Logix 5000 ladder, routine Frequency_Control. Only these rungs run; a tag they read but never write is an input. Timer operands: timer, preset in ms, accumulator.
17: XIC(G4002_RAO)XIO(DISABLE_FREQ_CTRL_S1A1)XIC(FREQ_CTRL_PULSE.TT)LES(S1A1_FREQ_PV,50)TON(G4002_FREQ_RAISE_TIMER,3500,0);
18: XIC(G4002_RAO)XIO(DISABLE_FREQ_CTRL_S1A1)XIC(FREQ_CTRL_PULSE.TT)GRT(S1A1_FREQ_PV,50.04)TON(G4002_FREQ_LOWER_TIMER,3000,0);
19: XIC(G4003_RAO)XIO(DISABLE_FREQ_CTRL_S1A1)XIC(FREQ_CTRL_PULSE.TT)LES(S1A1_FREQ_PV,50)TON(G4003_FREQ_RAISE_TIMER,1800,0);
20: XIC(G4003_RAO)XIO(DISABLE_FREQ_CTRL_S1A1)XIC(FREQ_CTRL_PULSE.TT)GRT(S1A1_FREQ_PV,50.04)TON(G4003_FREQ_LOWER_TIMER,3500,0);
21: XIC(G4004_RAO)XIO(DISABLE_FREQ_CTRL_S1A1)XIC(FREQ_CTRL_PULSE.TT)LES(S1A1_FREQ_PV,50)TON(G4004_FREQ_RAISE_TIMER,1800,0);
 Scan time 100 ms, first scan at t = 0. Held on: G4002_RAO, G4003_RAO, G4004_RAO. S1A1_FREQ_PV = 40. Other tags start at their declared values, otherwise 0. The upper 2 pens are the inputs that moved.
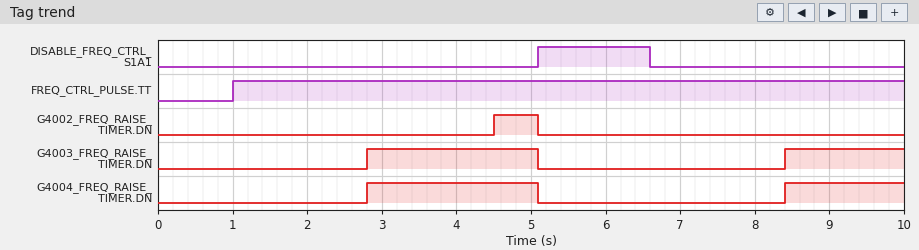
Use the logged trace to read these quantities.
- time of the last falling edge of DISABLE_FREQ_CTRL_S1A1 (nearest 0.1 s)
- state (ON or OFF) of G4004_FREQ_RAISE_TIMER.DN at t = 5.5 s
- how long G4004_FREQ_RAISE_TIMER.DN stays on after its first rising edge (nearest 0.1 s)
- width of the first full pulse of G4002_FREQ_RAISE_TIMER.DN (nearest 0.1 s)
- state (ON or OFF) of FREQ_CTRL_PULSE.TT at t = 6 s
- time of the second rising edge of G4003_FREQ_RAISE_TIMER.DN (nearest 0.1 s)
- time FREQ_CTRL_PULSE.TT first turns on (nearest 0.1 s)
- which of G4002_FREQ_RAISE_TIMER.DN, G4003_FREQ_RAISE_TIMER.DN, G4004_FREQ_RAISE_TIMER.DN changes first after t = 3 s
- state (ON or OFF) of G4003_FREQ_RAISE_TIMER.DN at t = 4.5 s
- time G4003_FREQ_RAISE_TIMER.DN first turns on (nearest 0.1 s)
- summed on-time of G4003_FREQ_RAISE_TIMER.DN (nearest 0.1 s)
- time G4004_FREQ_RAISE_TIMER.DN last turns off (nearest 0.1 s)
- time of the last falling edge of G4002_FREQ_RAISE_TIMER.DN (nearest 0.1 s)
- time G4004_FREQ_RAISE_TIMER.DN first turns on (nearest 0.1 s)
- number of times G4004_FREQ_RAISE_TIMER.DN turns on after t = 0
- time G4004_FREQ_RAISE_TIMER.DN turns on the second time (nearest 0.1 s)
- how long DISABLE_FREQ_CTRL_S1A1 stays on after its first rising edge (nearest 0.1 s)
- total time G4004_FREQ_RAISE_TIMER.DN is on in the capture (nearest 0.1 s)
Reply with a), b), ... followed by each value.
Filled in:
a) 6.6 s
b) OFF
c) 2.3 s
d) 0.6 s
e) ON
f) 8.4 s
g) 1.0 s
h) G4002_FREQ_RAISE_TIMER.DN
i) ON
j) 2.8 s
k) 3.9 s
l) 5.1 s
m) 5.1 s
n) 2.8 s
o) 2
p) 8.4 s
q) 1.5 s
r) 3.9 s
